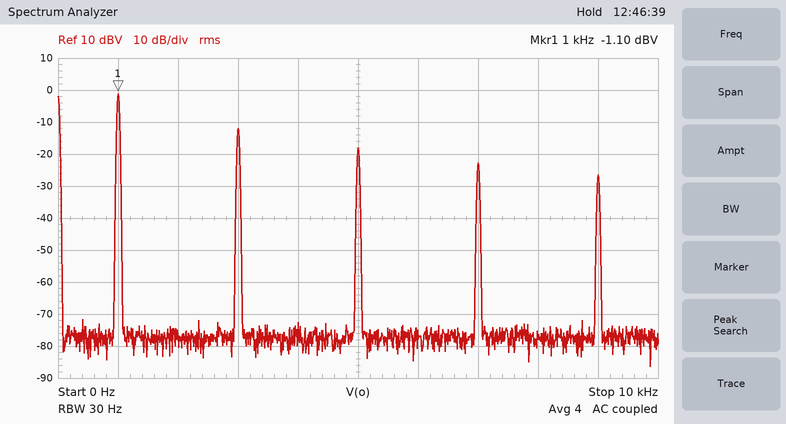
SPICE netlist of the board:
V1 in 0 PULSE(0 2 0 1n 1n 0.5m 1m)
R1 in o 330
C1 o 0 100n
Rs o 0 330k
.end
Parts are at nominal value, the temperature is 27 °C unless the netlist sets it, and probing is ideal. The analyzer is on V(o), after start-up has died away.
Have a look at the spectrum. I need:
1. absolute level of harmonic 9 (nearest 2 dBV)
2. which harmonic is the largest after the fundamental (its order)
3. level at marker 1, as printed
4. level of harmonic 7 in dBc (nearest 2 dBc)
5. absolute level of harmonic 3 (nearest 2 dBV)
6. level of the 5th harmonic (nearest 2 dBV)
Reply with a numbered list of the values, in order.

1. -26 dBV
2. 3
3. -1.10 dBV
4. -22 dBc
5. -12 dBV
6. -18 dBV
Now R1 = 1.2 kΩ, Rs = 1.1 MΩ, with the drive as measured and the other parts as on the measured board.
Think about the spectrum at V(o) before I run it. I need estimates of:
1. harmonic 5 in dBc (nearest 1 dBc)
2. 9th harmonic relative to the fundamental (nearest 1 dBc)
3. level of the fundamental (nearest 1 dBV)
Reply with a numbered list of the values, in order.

1. -24 dBc
2. -34 dBc
3. -3 dBV
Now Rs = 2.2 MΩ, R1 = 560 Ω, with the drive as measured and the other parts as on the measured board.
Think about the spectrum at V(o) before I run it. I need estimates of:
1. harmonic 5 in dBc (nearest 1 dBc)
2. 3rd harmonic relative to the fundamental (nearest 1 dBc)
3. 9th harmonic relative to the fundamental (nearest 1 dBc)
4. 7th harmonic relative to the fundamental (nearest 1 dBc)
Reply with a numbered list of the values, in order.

1. -20 dBc
2. -12 dBc
3. -29 dBc
4. -25 dBc
